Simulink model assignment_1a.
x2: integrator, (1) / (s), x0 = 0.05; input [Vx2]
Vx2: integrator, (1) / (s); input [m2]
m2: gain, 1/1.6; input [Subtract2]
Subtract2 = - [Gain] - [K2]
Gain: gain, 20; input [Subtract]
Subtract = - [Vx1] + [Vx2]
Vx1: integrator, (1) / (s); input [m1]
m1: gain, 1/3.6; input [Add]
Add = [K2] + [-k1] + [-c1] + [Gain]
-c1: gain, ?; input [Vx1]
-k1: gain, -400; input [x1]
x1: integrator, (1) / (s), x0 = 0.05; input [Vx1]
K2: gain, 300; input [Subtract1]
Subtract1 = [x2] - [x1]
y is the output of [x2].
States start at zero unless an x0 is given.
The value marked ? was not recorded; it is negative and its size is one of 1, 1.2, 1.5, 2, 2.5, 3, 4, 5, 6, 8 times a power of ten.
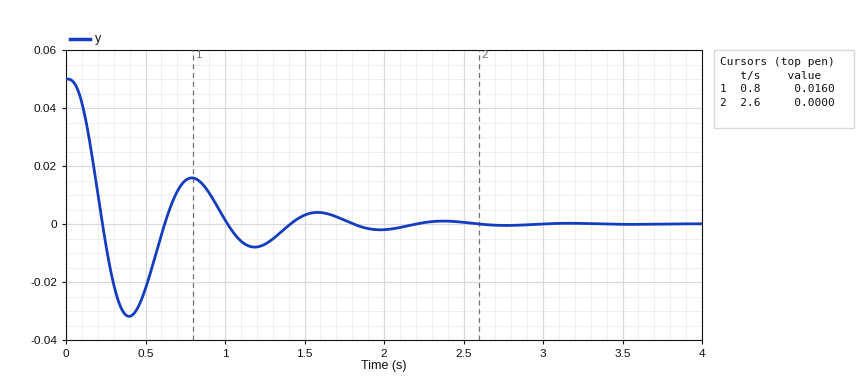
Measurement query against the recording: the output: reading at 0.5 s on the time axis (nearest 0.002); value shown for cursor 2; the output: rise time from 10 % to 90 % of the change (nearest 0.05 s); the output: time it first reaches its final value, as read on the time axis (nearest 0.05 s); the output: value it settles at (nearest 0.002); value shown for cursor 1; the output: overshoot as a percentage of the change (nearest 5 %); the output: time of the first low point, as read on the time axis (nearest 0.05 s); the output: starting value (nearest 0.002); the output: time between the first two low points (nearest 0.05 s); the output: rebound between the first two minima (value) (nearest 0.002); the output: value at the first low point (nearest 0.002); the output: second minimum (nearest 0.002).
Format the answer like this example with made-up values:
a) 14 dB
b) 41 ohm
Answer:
a) -0.022
b) 0.0000
c) 0.15 s
d) 0.25 s
e) 0.000
f) 0.0160
g) 65 %
h) 0.40 s
i) 0.050
j) 0.80 s
k) 0.016
l) -0.032
m) -0.008
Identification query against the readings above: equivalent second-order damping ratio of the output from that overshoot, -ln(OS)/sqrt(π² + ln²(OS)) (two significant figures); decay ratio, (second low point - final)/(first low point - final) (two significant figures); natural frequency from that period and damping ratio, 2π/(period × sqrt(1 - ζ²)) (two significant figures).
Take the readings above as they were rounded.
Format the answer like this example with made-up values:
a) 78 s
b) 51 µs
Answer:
a) 0.14
b) 0.25
c) 7.9 rad/s
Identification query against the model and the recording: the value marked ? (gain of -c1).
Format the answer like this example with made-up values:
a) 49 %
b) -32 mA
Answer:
a) -20
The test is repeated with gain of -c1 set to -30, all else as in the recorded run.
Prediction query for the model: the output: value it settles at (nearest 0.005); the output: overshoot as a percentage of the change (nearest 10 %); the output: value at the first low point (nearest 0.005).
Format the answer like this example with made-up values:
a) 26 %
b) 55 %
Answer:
a) 0.000
b) 50 %
c) -0.025
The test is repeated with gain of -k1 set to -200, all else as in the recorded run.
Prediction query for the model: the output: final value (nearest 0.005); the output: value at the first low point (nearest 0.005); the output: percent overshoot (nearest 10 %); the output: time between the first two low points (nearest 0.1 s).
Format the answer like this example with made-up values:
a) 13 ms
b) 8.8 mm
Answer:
a) 0.000
b) -0.020
c) 40 %
d) 1.1 s
